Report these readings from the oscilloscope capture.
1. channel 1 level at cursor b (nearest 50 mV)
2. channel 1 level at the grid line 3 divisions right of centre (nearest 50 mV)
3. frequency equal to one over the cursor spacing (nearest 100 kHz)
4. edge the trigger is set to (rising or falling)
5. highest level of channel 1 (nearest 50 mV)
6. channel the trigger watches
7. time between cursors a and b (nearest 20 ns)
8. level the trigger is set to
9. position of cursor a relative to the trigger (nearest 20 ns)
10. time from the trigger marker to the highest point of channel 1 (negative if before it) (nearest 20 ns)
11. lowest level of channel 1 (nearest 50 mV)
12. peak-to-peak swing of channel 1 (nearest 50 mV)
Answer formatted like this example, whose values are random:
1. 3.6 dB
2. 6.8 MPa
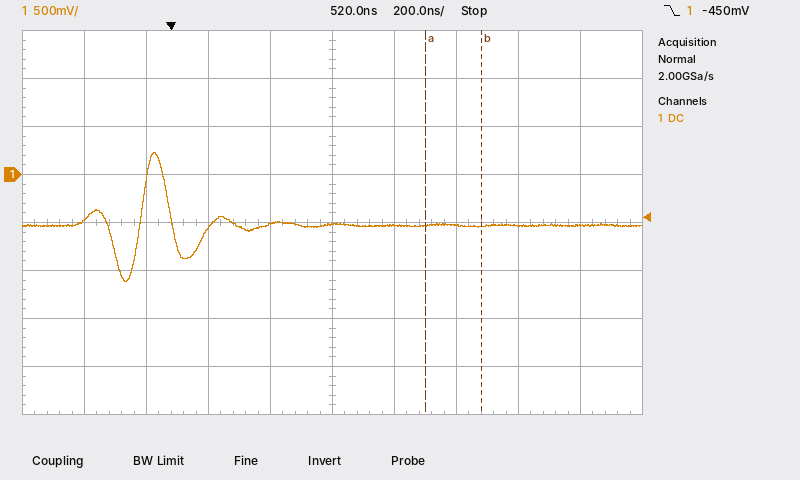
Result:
1. -550 mV
2. -550 mV
3. 5.6 MHz
4. falling
5. 250 mV
6. channel 1
7. 180 ns
8. -450 mV
9. +820 ns
10. -60 ns
11. -1.10 V
12. 1.35 V
